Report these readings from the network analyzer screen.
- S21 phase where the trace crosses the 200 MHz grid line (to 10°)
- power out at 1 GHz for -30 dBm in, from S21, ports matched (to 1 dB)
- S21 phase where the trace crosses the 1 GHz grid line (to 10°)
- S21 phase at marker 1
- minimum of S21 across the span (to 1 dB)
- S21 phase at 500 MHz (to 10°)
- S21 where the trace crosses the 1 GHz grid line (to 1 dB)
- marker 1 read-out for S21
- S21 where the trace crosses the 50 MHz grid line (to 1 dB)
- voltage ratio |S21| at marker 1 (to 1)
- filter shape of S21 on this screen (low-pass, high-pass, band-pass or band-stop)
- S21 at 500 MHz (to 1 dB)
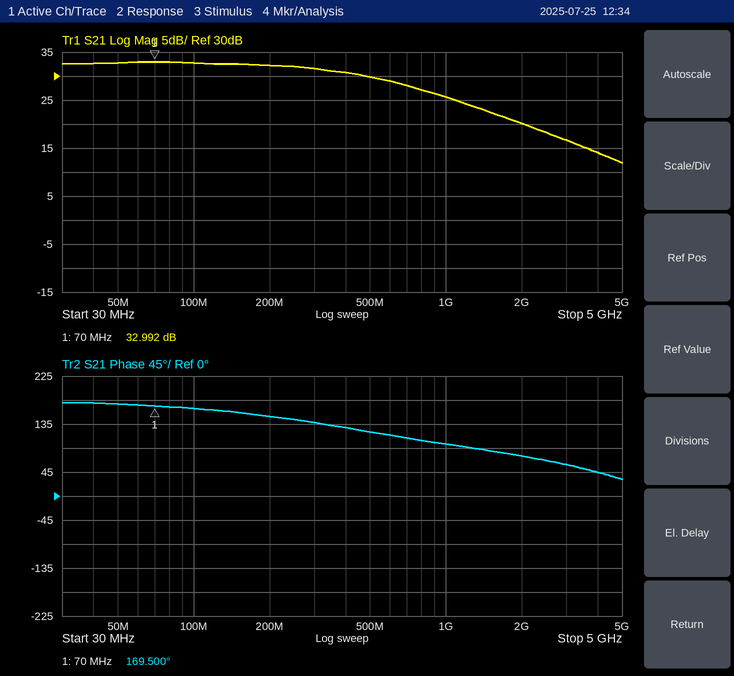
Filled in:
150°
-4 dBm
100°
169.500°
12 dB
120°
26 dB
32.992 dB
33 dB
45
low-pass
30 dB
